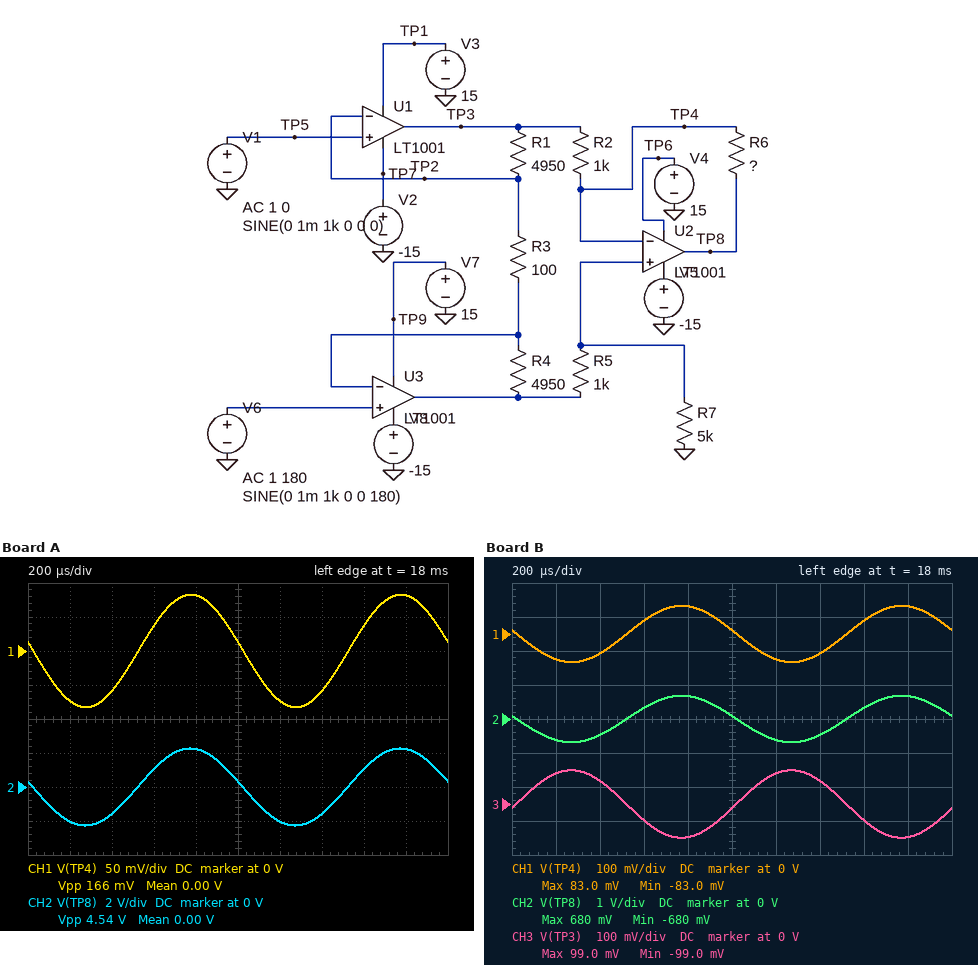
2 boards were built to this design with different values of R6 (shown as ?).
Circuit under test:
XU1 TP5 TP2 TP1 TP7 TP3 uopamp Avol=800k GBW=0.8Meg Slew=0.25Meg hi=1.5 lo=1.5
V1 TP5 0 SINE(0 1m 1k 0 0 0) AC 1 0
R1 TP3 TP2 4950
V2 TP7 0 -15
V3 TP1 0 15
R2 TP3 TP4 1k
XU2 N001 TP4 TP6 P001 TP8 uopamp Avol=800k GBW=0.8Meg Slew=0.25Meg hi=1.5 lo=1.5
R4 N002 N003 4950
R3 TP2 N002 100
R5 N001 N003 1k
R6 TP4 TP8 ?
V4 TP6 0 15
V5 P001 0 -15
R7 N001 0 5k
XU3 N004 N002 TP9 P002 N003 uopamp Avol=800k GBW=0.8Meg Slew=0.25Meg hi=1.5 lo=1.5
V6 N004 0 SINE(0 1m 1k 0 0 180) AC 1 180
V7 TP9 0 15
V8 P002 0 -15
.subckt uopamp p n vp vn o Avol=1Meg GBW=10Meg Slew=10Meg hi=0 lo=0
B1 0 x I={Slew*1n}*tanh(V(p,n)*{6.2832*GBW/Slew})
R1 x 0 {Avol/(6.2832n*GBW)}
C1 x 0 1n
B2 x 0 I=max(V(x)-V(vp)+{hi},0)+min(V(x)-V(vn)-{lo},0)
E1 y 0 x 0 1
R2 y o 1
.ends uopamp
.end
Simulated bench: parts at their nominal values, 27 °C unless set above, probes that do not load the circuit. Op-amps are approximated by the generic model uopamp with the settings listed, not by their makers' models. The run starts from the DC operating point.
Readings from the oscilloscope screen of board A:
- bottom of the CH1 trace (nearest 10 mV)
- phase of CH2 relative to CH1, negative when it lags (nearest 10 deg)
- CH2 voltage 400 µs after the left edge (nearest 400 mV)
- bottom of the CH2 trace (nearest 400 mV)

-80 mV
0 deg
-1.6 V
-2.4 V
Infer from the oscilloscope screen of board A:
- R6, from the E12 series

12 kΩ
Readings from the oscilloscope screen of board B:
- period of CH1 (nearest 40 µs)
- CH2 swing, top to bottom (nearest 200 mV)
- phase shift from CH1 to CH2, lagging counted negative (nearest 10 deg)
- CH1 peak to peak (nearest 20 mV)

1.00 ms
1.4 V
0 deg
160 mV
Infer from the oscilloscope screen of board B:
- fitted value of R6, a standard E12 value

3.3 kΩ
